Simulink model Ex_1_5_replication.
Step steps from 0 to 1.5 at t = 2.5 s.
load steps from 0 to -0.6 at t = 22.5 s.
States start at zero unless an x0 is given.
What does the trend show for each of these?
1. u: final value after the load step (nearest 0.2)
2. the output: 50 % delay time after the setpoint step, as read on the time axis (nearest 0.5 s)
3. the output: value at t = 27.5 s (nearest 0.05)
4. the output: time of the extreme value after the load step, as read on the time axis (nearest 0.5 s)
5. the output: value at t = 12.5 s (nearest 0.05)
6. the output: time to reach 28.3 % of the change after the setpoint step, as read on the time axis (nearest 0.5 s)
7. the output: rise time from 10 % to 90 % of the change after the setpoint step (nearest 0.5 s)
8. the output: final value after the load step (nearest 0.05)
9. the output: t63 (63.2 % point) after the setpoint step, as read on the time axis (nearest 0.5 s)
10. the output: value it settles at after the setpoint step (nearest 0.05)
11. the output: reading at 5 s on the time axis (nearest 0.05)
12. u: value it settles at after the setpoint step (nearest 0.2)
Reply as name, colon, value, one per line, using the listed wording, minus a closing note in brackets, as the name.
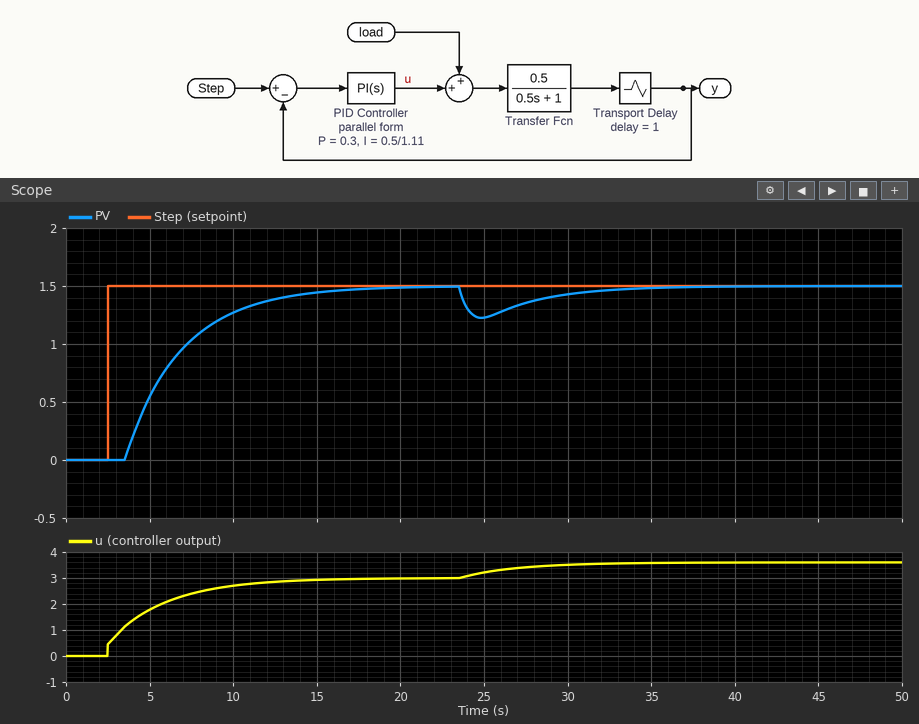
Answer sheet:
u: final value after the load step: 3.6
the output: 50 % delay time after the setpoint step, as read on the time axis: 6.0 s
the output: value at t = 27.5 s: 1.35
the output: time of the extreme value after the load step, as read on the time axis: 25.0 s
the output: value at t = 12.5 s: 1.40
the output: time to reach 28.3 % of the change after the setpoint step, as read on the time axis: 4.5 s
the output: rise time from 10 % to 90 % of the change after the setpoint step: 7.5 s
the output: final value after the load step: 1.50
the output: t63 (63.2 % point) after the setpoint step, as read on the time axis: 7.0 s
the output: value it settles at after the setpoint step: 1.50
the output: reading at 5 s on the time axis: 0.55
u: value it settles at after the setpoint step: 3.0
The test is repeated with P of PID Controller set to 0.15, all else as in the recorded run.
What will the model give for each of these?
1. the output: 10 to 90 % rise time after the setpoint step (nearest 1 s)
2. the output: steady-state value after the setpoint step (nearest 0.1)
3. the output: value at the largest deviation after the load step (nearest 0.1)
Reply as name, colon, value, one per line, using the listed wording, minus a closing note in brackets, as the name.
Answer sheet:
the output: 10 to 90 % rise time after the setpoint step: 7 s
the output: steady-state value after the setpoint step: 1.5
the output: value at the largest deviation after the load step: 1.2
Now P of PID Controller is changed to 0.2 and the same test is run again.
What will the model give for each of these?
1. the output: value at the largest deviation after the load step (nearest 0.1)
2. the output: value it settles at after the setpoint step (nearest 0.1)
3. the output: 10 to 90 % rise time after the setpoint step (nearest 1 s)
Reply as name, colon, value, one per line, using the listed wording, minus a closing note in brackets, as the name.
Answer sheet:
the output: value at the largest deviation after the load step: 1.2
the output: value it settles at after the setpoint step: 1.5
the output: 10 to 90 % rise time after the setpoint step: 7 s
